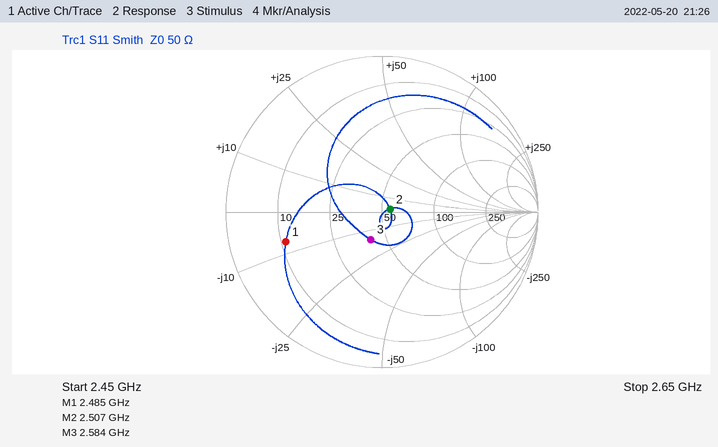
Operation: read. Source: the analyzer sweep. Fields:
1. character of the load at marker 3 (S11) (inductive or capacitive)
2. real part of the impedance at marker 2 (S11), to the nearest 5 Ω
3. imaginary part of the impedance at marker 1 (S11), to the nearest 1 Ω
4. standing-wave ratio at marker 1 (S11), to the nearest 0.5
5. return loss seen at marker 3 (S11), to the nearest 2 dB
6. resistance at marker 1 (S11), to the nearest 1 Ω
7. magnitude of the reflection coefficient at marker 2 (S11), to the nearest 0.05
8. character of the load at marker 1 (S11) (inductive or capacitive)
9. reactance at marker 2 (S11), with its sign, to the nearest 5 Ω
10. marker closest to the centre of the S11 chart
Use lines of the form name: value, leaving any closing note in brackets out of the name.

character of the load at marker 3 (S11): capacitive
real part of the impedance at marker 2 (S11), to the nearest 5 Ω: 55 Ω
imaginary part of the impedance at marker 1 (S11), to the nearest 1 Ω: -7 Ω
standing-wave ratio at marker 1 (S11), to the nearest 0.5: 4.5
return loss seen at marker 3 (S11), to the nearest 2 dB: 14 dB
resistance at marker 1 (S11), to the nearest 1 Ω: 11 Ω
magnitude of the reflection coefficient at marker 2 (S11), to the nearest 0.05: 0.05
character of the load at marker 1 (S11): capacitive
reactance at marker 2 (S11), with its sign, to the nearest 5 Ω: 0 Ω
marker closest to the centre of the S11 chart: marker 2
